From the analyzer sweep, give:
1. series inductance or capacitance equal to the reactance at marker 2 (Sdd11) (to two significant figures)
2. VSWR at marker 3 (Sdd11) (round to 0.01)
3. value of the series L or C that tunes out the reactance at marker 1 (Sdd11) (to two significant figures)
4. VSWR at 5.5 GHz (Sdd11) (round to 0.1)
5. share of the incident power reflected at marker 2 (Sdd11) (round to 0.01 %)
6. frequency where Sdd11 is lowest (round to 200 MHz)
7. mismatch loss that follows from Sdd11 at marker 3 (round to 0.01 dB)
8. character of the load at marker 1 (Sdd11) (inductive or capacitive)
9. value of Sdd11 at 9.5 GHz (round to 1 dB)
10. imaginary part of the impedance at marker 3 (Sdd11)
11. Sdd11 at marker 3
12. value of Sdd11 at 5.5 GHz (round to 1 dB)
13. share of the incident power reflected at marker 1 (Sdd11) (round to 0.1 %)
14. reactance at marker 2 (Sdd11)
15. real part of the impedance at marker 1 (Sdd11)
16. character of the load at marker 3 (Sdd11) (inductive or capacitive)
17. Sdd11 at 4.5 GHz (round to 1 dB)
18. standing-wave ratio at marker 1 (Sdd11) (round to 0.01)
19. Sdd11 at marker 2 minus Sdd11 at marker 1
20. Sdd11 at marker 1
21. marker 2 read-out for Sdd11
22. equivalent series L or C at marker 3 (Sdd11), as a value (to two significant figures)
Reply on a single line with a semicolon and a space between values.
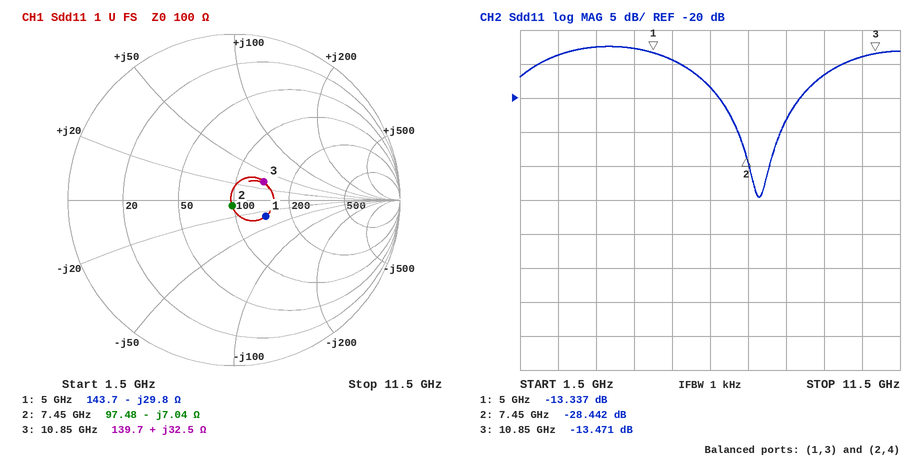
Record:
3.0 pF; 1.54; 950 pH; 1.5; 0.14 %; 7.8 GHz; 0.20 dB; capacitive; -17 dB; +32.5 Ω; -13.471 dB; -14 dB; 4.6 %; -7.04 Ω; 143.7 Ω; inductive; -13 dB; 1.55; -15.105 dB; -13.337 dB; -28.442 dB; 480 pH
